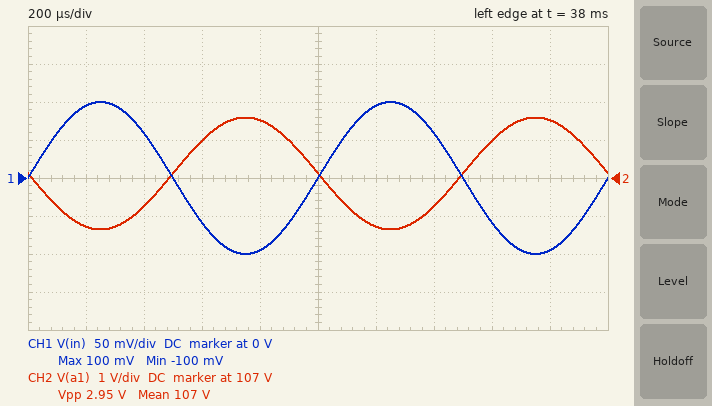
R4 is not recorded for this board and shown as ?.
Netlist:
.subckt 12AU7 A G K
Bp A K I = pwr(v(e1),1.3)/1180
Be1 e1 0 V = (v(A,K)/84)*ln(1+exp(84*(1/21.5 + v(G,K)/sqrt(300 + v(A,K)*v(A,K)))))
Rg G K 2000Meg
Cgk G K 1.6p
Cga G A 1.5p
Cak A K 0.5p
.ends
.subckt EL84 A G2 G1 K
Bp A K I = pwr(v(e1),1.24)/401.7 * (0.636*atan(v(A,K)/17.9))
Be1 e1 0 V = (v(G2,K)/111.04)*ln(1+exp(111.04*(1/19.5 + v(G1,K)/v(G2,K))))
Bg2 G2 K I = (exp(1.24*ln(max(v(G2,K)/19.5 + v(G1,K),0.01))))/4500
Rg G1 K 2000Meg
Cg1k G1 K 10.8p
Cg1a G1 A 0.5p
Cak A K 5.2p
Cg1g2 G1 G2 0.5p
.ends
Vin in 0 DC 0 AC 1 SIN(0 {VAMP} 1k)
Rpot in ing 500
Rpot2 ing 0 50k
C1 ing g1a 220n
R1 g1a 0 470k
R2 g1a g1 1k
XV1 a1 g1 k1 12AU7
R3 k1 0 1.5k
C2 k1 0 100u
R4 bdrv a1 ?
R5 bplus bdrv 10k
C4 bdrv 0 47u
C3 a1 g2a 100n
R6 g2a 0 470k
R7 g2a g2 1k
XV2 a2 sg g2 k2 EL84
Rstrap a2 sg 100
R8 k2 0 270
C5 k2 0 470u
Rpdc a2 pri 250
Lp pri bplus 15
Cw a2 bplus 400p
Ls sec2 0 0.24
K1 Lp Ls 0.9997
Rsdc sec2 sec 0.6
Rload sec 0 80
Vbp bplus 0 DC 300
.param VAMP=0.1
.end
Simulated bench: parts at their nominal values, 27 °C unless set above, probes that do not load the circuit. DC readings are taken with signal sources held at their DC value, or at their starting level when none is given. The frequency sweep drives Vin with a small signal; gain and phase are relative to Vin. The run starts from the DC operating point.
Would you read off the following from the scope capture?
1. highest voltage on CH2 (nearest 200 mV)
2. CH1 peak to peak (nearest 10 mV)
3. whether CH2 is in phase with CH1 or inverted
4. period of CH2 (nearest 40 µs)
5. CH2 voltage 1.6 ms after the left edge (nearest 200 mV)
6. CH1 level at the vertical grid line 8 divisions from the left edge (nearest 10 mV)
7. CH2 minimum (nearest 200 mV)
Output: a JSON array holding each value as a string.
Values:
["108.6 V", "200 mV", "inverted", "1.00 ms", "108.0 V", "-60 mV", "105.6 V"]
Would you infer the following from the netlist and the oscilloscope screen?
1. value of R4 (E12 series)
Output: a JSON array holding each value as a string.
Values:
["82 kΩ"]
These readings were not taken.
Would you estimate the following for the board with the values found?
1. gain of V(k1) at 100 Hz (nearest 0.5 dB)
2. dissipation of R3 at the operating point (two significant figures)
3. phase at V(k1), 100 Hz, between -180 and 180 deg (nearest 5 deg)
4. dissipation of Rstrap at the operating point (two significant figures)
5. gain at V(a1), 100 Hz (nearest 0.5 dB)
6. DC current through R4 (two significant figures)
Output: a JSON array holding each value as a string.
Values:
["-49.5 dB", "6.6 mW", "-90 deg", "570 µW", "23.5 dB", "2.1 mA"]
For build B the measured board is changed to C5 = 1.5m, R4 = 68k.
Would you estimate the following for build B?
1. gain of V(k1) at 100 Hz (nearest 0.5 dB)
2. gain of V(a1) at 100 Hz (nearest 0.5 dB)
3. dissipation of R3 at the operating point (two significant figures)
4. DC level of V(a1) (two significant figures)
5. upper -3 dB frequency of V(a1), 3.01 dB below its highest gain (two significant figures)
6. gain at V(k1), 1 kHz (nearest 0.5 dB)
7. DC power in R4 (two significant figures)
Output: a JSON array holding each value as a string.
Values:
["-48.5 dB", "23.0 dB", "8.2 mW", "120 V", "570 kHz", "-68.5 dB", "370 mW"]
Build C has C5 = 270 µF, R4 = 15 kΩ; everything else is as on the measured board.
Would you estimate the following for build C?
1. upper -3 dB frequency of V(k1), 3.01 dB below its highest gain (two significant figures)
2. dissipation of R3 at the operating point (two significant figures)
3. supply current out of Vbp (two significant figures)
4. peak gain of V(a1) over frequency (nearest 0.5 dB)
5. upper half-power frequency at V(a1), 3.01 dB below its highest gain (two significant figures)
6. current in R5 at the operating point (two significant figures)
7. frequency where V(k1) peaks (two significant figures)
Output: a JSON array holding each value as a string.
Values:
["4.5 Hz", "25 mW", "33 mA", "19.0 dB", "1.1 MHz", "4.1 mA", "1.8 Hz"]
